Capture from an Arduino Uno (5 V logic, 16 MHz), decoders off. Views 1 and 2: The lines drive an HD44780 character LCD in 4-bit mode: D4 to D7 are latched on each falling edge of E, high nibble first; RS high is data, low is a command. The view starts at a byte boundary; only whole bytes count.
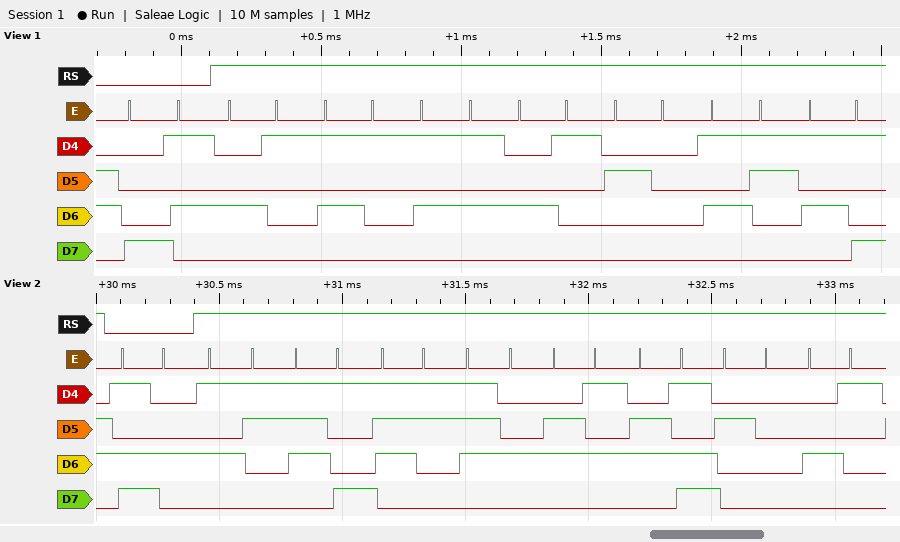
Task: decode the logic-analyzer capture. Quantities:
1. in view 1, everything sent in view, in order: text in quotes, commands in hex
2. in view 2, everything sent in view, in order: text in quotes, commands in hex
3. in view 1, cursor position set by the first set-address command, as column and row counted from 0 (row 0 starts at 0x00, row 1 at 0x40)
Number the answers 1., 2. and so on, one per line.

1. 0x85 "AQUA SY"
2. 0xD4 "System A"
3. column 5, row 0
